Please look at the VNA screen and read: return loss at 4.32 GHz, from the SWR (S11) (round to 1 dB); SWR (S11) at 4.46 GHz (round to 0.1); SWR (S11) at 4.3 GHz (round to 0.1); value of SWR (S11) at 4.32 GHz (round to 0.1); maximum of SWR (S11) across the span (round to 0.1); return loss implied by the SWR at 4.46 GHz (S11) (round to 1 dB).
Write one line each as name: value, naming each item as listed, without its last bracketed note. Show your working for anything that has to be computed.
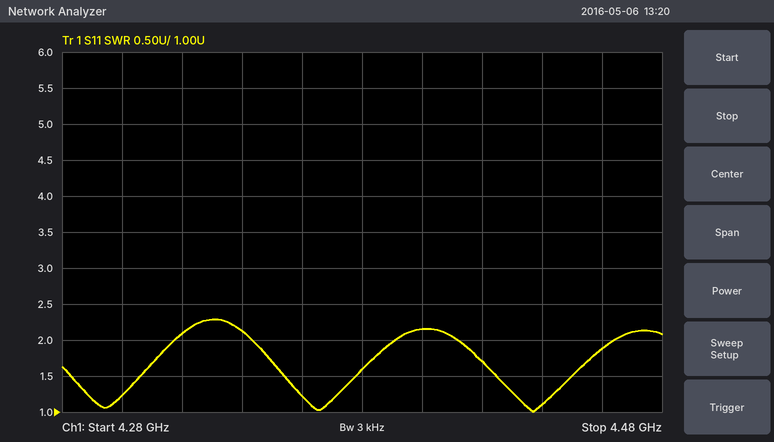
return loss at 4.32 GHz, from the SWR (S11): −20 log10((2.1 − 1)/(2.1 + 1)) ≈ 9 dB
SWR (S11) at 4.46 GHz: 1.9
SWR (S11) at 4.3 GHz: 1.2
value of SWR (S11) at 4.32 GHz: 2.1
maximum of SWR (S11) across the span: 2.3
return loss implied by the SWR at 4.46 GHz (S11): −20 log10((1.9 − 1)/(1.9 + 1)) ≈ 10 dB
